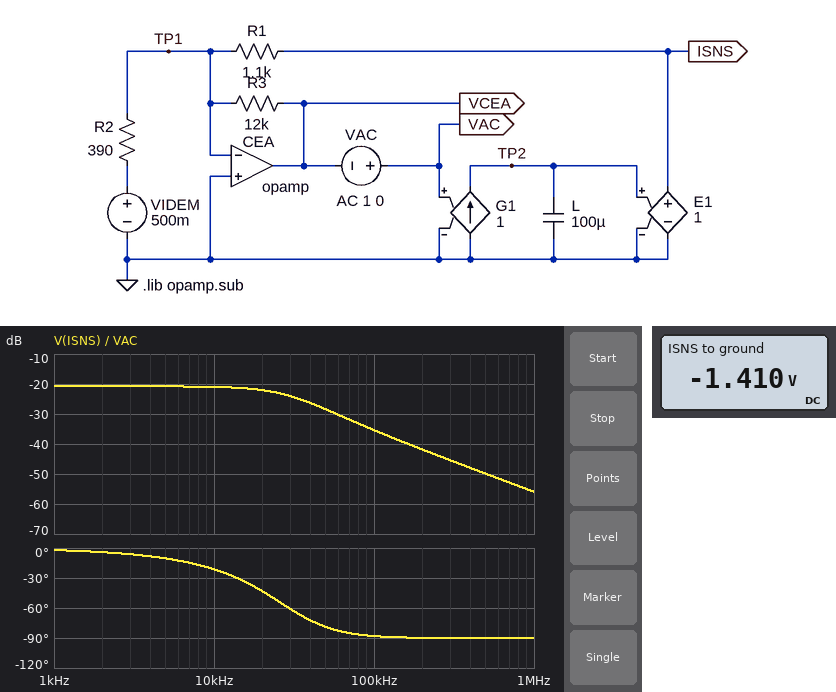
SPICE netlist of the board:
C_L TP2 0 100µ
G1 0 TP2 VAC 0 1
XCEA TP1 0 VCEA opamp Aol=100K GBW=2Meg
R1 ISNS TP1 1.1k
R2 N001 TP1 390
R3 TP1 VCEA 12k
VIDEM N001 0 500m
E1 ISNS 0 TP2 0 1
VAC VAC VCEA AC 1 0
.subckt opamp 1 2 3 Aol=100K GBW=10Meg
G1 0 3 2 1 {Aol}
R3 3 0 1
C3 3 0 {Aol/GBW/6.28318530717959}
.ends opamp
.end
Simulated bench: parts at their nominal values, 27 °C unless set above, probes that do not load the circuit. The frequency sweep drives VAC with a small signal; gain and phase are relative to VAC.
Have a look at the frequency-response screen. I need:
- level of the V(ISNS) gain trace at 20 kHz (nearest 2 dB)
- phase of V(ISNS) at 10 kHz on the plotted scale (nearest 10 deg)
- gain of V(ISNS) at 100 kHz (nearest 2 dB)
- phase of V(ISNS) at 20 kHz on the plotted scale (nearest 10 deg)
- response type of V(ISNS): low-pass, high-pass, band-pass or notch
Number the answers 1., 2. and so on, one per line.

1. -22 dB
2. -20 deg
3. -36 dB
4. -40 deg
5. low-pass
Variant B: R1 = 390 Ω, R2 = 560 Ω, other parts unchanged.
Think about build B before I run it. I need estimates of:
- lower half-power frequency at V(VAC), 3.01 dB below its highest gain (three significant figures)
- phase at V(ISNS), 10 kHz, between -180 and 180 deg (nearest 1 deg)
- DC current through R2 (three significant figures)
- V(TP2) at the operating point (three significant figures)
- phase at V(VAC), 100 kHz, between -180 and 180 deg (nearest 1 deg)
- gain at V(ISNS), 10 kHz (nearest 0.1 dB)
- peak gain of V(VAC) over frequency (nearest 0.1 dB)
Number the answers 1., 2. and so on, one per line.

1. 32.5 kHz
2. 3 deg
3. 893 µA
4. -348 mV
5. 4 deg
6. -29.2 dB
7. 3.9 dB
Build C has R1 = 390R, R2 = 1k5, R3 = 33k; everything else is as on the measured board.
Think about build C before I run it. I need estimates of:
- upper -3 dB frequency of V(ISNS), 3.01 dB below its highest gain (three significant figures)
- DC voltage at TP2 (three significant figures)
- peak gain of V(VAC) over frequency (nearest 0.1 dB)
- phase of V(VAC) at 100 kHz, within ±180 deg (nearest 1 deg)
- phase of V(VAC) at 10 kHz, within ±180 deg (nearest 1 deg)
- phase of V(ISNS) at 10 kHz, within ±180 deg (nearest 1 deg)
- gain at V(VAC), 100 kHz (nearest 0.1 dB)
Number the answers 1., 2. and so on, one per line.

1. 59.8 kHz
2. -130 mV
3. 9.3 dB
4. 3 deg
5. 114 deg
6. 24 deg
7. 2.4 dB
